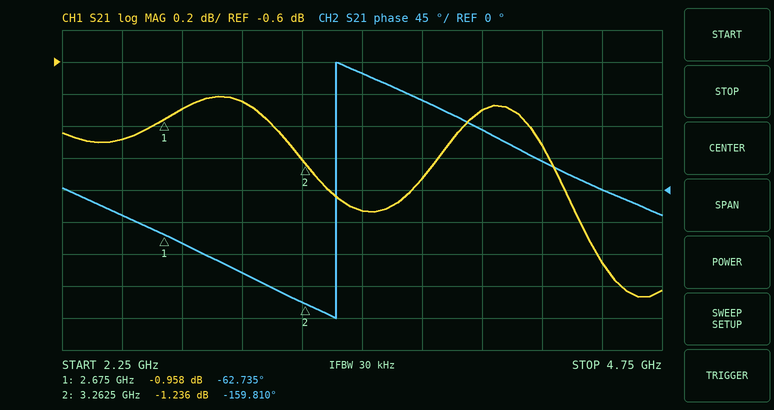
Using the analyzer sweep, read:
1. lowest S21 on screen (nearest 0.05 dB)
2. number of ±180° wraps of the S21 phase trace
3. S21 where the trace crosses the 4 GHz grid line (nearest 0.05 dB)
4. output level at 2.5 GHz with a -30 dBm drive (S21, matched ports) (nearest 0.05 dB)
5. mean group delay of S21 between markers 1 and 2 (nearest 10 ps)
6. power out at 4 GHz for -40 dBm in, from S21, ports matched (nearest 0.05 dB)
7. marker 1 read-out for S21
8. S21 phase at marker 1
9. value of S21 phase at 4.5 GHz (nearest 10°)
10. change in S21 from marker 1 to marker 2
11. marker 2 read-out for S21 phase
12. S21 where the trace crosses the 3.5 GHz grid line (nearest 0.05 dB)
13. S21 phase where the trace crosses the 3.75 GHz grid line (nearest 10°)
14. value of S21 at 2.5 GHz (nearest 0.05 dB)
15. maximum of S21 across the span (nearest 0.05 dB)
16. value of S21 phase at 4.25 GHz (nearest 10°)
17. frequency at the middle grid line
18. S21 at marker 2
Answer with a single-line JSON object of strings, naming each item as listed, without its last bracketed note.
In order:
{"lowest S21 on screen": "-2.05 dB", "number of ±180° wraps of the S21 phase trace": "1", "S21 where the trace crosses the 4 GHz grid line": "-0.90 dB", "output level at 2.5 GHz with a -30 dBm drive (S21, matched ports)": "-31.10 dBm", "mean group delay of S21 between markers 1 and 2": "460 ps", "power out at 4 GHz for -40 dBm in, from S21, ports matched": "-40.90 dBm", "marker 1 read-out for S21": "-0.958 dB", "S21 phase at marker 1": "-62.735°", "value of S21 phase at 4.5 GHz": "0°", "change in S21 from marker 1 to marker 2": "-0.278 dB", "marker 2 read-out for S21 phase": "-159.810°", "S21 where the trace crosses the 3.5 GHz grid line": "-1.55 dB", "S21 phase where the trace crosses the 3.75 GHz grid line": "130°", "value of S21 at 2.5 GHz": "-1.10 dB", "maximum of S21 across the span": "-0.80 dB", "value of S21 phase at 4.25 GHz": "40°", "frequency at the middle grid line": "3.5 GHz", "S21 at marker 2": "-1.236 dB"}
